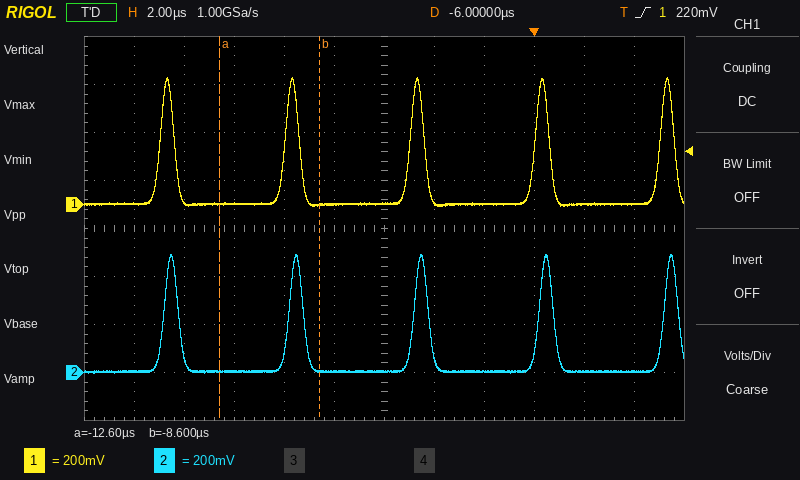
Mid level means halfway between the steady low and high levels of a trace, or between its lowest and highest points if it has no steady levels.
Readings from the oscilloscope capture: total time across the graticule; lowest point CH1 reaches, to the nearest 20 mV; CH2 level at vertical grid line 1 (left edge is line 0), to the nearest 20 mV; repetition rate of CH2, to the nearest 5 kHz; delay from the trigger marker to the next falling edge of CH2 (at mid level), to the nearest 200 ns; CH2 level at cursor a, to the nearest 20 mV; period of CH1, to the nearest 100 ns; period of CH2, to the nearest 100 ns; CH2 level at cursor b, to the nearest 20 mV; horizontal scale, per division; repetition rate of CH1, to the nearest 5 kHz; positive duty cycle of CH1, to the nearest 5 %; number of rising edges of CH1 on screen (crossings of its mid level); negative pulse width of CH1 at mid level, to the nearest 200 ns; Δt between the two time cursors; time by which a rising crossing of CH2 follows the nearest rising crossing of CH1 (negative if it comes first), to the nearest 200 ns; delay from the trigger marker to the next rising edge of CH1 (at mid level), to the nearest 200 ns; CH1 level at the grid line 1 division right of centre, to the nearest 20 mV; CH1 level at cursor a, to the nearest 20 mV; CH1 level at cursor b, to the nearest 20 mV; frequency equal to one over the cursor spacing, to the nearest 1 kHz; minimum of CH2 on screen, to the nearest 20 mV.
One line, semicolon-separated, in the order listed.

24 µs; 0 mV; 0 mV; 200 kHz; 800 ns; 0 mV; 5.0 µs; 5.0 µs; 0 mV; 2 µs; 200 kHz; 10 %; 5; 4.4 µs; 4.0 µs; +200 ns; 5.0 µs; 20 mV; 0 mV; 0 mV; 250 kHz; 0 mV
